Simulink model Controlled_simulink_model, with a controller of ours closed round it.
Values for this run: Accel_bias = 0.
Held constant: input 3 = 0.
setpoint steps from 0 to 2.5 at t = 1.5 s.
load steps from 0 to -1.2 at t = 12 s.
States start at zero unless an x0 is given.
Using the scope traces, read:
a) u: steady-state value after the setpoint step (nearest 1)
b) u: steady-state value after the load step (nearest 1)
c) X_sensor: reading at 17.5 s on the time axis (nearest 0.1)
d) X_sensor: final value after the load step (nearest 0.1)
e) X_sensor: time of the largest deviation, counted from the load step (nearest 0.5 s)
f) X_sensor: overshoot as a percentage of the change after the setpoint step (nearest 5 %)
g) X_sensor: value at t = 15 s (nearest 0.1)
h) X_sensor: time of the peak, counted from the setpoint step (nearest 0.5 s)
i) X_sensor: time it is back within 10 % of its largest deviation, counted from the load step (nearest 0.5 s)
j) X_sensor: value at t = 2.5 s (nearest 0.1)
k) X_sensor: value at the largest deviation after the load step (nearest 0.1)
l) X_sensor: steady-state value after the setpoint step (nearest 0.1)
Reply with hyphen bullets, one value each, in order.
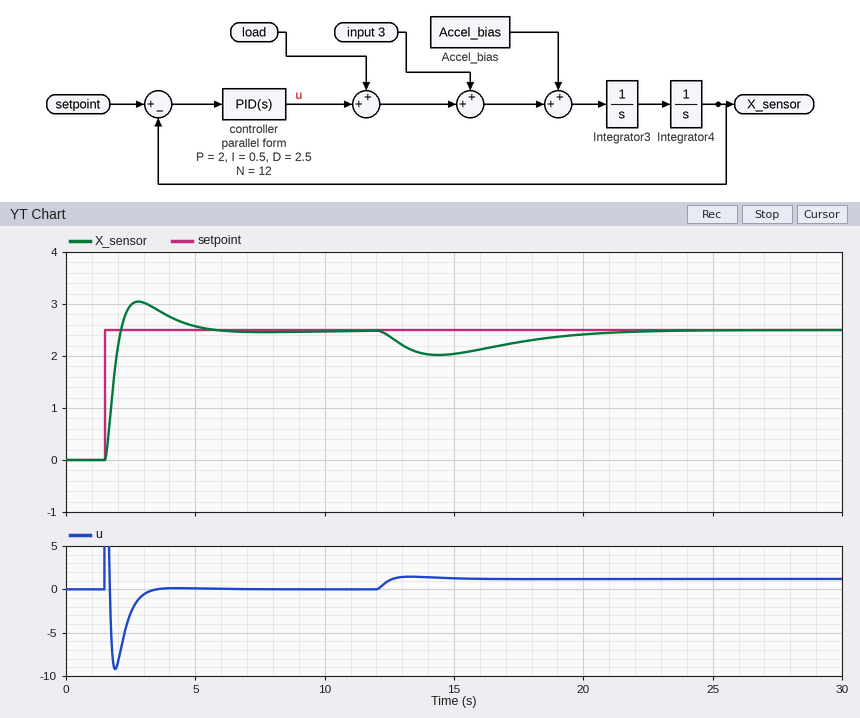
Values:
- 0
- 1
- 2.3
- 2.5
- 2.5 s
- 20 %
- 2.0
- 1.5 s
- 9.5 s
- 3.0
- 2.0
- 2.5
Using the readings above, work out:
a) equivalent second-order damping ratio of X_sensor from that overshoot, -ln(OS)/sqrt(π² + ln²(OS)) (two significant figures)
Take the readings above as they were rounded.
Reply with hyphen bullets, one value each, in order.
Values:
- 0.46
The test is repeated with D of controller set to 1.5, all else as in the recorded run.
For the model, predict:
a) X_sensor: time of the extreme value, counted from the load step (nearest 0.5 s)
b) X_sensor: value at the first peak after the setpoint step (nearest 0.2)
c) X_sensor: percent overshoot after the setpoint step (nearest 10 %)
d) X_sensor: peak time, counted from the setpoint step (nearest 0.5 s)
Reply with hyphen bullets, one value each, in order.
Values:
- 2.0 s
- 3.4
- 40 %
- 1.5 s
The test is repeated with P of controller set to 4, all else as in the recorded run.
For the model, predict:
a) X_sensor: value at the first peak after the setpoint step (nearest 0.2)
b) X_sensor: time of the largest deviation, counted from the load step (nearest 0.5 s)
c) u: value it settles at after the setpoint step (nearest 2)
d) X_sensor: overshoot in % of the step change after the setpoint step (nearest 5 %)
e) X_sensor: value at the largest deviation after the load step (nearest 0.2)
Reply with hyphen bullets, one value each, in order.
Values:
- 3.2
- 1.5 s
- 0
- 30 %
- 2.2
